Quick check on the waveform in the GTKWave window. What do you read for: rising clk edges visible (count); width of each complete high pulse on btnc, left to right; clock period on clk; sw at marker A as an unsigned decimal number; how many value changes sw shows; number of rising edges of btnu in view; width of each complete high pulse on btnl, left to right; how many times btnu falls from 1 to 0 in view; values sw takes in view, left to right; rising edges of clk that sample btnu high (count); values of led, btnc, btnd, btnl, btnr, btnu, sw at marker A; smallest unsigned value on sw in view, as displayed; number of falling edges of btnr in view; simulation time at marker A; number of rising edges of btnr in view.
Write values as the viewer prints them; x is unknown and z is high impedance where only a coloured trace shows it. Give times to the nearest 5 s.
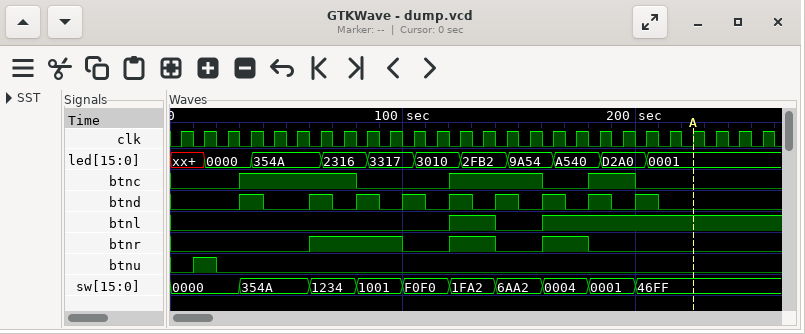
26
50 s, 40 s, 20 s
10 s
18175
9
1
20 s
1
0000, 354A, 1234, 1001, F0F0, 1FA2, 6AA2, 0004, 0001, 46FF
1
led=0001, btnc=0, btnd=0, btnl=1, btnr=0, btnu=0, sw=46FF
0000
3
225 s
3
